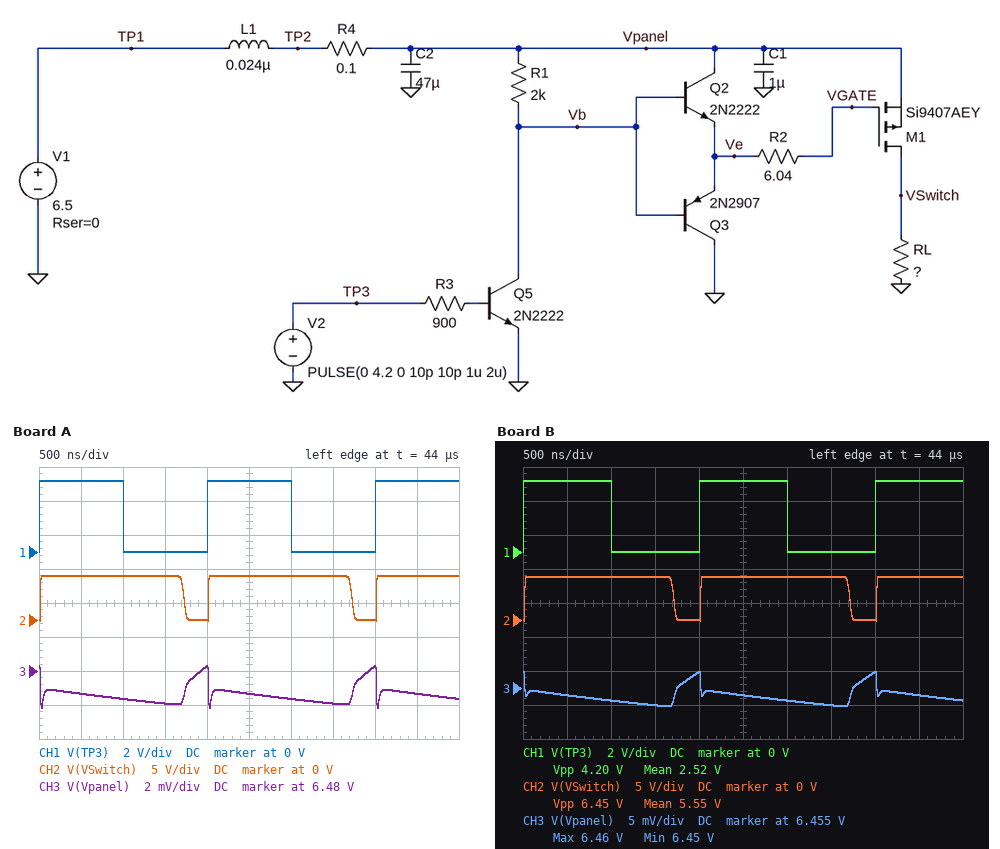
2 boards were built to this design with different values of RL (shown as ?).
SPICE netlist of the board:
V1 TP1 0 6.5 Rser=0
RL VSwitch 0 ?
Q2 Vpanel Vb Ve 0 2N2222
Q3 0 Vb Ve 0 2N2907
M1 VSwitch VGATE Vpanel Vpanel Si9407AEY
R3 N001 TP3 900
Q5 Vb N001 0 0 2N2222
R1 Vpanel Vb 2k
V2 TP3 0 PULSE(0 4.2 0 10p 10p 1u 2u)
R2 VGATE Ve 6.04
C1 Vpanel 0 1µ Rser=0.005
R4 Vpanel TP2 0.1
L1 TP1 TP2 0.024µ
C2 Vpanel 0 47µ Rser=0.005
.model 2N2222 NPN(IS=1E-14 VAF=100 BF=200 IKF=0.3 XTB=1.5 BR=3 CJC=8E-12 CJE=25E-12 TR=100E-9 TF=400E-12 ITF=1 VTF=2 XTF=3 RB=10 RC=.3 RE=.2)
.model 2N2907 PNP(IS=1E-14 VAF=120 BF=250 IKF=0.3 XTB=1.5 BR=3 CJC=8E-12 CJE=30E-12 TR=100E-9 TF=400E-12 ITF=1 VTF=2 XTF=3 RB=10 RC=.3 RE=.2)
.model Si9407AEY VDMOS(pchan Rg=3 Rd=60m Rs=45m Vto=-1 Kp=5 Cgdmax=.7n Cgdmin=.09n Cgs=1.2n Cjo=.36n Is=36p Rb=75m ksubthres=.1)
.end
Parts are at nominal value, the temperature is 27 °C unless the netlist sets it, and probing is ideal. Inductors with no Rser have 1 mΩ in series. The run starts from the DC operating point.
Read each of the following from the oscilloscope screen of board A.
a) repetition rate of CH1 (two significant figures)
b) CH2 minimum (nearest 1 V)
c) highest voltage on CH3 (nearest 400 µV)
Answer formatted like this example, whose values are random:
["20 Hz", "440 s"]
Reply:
["500 kHz", "0 V", "6.4804 V"]
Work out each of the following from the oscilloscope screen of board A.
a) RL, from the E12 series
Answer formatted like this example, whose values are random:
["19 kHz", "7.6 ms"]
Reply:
["27 Ω"]
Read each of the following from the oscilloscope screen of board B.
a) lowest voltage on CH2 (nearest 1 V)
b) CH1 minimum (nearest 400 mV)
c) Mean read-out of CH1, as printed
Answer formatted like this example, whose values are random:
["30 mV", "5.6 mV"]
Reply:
["0 V", "0 V", "2.52 V"]
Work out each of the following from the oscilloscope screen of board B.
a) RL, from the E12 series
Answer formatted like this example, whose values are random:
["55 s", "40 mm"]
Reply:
["12 Ω"]
